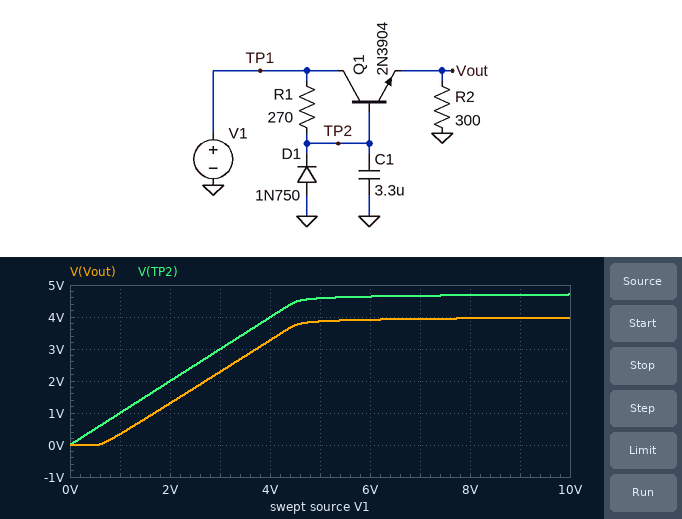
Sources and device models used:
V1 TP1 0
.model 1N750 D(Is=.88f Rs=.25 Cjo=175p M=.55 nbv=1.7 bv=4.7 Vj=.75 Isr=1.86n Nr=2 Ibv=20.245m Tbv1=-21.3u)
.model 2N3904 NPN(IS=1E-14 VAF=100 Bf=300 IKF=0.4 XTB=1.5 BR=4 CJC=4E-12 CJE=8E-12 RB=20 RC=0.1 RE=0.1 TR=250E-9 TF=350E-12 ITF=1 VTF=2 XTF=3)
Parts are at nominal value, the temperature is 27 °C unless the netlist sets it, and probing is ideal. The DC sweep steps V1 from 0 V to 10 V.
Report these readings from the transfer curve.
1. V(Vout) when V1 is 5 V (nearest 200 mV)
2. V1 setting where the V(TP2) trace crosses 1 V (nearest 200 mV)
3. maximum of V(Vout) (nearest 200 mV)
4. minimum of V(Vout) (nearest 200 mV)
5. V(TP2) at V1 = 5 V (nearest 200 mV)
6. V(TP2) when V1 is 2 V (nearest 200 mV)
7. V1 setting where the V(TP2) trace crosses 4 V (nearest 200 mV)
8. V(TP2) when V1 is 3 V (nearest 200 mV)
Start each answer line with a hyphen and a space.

- 3.8 V
- 1.0 V
- 4.0 V
- 0 V
- 4.6 V
- 2.0 V
- 4.0 V
- 3.0 V
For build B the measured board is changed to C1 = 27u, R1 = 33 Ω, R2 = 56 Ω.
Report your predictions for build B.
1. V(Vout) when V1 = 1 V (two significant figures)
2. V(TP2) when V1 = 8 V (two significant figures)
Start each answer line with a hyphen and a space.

- 300 mV
- 4.8 V
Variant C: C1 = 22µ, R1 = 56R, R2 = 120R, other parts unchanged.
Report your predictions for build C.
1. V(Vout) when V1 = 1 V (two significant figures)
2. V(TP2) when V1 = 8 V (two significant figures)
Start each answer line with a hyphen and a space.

- 320 mV
- 4.8 V
